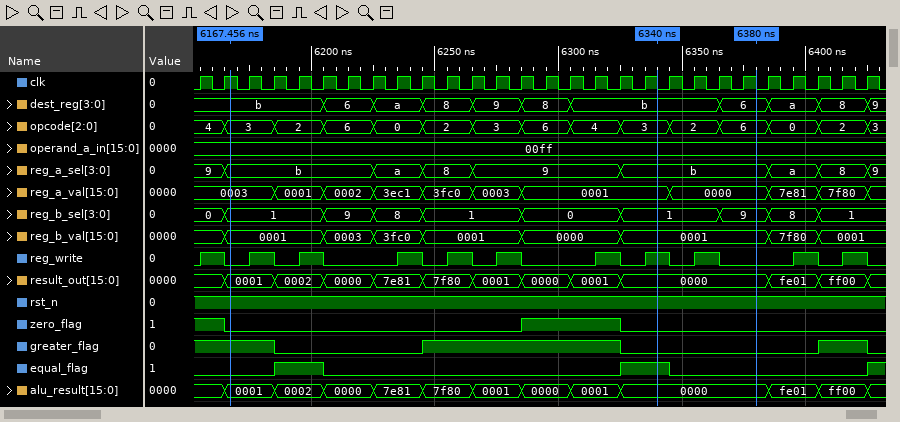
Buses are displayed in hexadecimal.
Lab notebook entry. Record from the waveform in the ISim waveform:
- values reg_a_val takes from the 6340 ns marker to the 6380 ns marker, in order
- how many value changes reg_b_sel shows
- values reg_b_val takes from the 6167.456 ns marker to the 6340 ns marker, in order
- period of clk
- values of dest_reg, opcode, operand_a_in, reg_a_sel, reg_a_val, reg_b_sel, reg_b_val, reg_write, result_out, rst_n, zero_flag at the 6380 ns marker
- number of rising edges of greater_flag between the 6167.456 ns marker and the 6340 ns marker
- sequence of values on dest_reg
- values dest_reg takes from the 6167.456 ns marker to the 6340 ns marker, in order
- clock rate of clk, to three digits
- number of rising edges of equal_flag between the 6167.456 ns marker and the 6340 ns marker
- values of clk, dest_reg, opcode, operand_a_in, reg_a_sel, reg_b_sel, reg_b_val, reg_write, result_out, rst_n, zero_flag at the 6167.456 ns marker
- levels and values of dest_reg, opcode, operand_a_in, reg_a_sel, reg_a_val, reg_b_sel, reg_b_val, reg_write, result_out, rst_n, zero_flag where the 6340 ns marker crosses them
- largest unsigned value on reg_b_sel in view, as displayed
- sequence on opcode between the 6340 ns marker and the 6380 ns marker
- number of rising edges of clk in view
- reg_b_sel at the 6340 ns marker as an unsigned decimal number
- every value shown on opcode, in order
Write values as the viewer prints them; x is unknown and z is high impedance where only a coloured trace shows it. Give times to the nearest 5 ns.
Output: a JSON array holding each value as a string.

["0001, 0000", "9", "0001, 0003, 3fc0, 0001, 0000, 0001", "10 ns", "dest_reg=6, opcode=6, operand_a_in=00ff, reg_a_sel=b, reg_a_val=0000, reg_b_sel=9, reg_b_val=0001, reg_write=0, result_out=0000, rst_n=1, zero_flag=0", "1", "b, 6, a, 8, 9, 8, b, 6, a, 8, 9", "b, 6, a, 8, 9, 8, b", "100 MHz", "2", "clk=1, dest_reg=b, opcode=3, operand_a_in=00ff, reg_a_sel=b, reg_b_sel=1, reg_b_val=0001, reg_write=0, result_out=0001, rst_n=1, zero_flag=0", "dest_reg=b, opcode=3, operand_a_in=00ff, reg_a_sel=b, reg_a_val=0001, reg_b_sel=1, reg_b_val=0001, reg_write=1, result_out=0000, rst_n=1, zero_flag=0", "9", "3, 2, 6", "28", "1", "4, 3, 2, 6, 0, 2, 3, 6, 4, 3, 2, 6, 0, 2, 3"]
